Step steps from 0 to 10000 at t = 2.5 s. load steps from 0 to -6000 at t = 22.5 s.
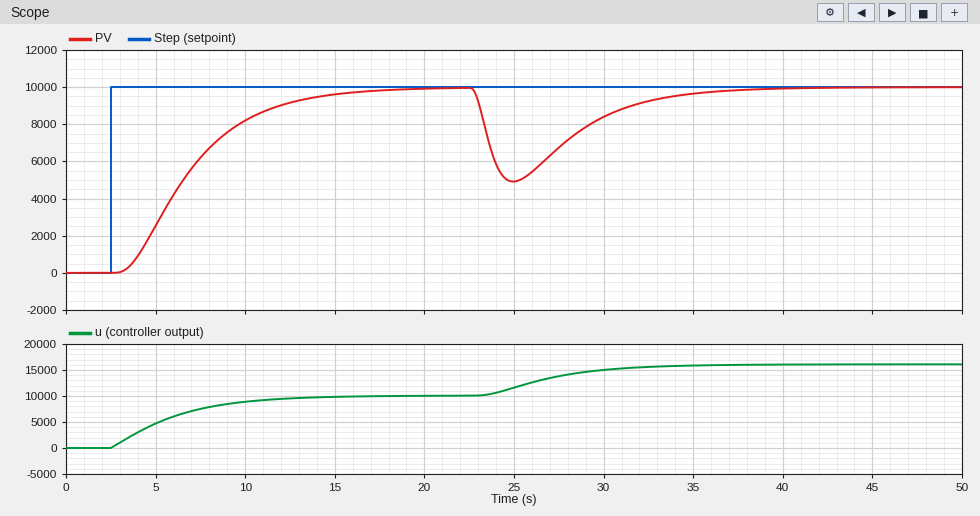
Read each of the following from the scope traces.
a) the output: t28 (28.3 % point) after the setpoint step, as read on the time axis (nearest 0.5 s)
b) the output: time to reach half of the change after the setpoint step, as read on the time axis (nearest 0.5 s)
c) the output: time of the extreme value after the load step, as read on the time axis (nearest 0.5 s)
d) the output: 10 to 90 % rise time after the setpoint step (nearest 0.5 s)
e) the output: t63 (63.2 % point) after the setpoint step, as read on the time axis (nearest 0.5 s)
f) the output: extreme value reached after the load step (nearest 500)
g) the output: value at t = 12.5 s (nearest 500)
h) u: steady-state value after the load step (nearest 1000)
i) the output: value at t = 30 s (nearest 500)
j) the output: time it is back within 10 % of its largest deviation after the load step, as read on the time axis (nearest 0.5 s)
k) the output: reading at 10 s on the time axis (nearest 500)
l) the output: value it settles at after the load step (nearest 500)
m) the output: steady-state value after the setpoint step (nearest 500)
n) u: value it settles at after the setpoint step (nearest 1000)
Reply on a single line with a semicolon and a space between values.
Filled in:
5.0 s; 6.5 s; 25.0 s; 8.0 s; 7.5 s; 5000; 9000; 16000; 8500; 34.0 s; 8000; 10000; 10000; 10000
